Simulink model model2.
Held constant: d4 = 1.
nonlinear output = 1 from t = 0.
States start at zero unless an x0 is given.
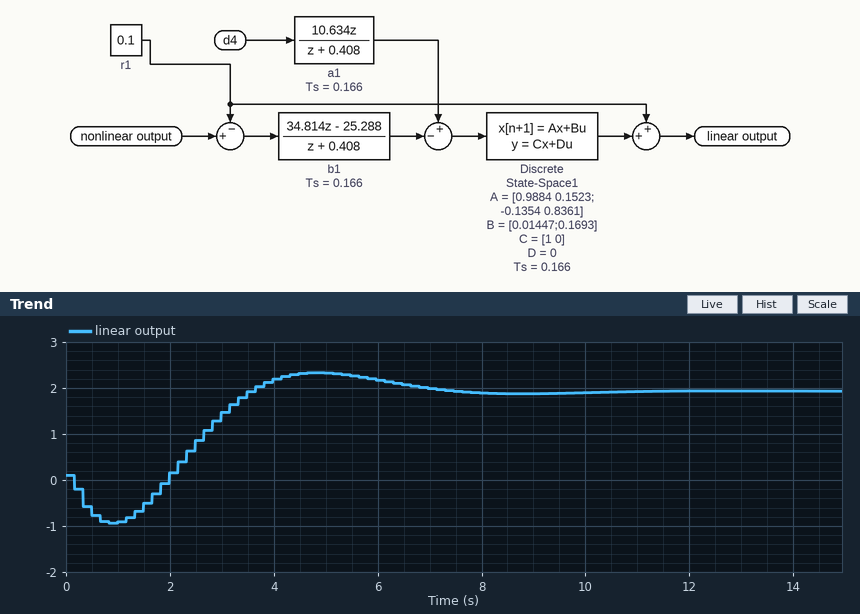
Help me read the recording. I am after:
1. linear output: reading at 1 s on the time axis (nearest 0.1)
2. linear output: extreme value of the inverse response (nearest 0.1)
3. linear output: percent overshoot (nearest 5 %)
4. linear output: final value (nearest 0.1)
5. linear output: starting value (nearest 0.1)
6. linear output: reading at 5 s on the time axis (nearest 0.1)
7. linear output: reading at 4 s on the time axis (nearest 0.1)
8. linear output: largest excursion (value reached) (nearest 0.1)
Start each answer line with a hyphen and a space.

- -0.9
- -0.9
- 20 %
- 1.9
- 0.1
- 2.3
- 2.2
- 2.3
